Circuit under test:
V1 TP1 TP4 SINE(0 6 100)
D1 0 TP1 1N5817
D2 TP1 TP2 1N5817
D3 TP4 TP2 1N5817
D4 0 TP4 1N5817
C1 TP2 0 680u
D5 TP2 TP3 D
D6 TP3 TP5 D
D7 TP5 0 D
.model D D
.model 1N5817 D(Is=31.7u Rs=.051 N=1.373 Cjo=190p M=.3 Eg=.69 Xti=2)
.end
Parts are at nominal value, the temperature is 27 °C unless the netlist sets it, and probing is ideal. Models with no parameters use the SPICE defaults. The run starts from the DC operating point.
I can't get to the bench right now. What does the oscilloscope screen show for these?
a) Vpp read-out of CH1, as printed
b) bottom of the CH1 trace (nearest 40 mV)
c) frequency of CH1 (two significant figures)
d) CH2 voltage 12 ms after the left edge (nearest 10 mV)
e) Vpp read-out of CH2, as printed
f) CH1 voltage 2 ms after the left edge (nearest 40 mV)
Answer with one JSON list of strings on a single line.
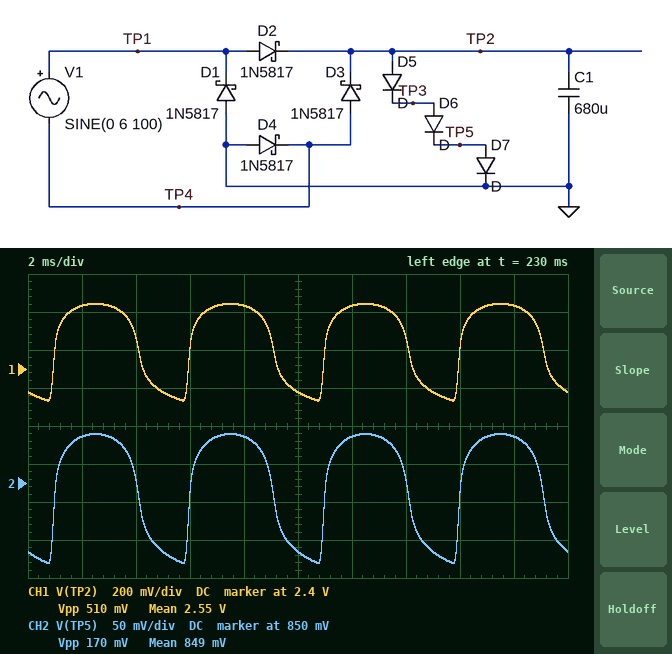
["510 mV", "2.24 V", "200 Hz", "910 mV", "170 mV", "2.72 V"]
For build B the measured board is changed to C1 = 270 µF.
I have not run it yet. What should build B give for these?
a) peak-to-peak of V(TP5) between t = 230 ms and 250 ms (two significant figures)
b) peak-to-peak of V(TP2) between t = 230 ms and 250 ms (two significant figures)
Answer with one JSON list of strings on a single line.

["190 mV", "580 mV"]
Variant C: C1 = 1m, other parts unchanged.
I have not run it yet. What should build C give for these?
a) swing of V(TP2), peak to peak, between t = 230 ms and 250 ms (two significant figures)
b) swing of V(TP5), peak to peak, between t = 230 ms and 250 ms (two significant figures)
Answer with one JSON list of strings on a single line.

["480 mV", "160 mV"]
